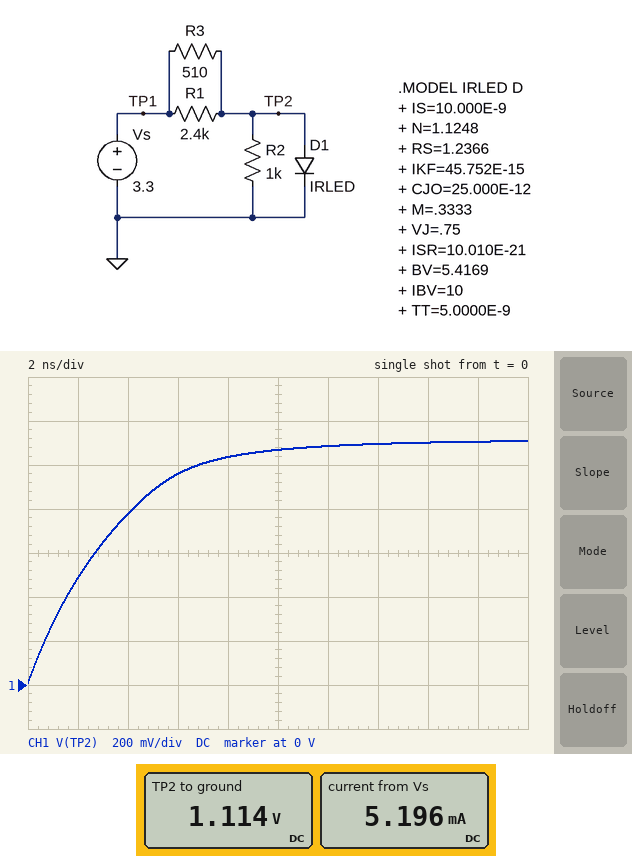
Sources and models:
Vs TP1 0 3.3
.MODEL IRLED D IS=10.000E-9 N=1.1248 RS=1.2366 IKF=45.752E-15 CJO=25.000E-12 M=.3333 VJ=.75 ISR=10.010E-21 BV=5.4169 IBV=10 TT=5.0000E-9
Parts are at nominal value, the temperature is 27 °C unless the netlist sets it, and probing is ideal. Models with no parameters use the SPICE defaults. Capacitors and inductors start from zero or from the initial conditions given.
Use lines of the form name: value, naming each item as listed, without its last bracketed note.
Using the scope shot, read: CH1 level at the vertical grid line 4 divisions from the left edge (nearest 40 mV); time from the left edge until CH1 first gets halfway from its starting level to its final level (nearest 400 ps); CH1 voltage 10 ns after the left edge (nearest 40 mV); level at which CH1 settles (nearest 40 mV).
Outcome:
CH1 level at the vertical grid line 4 divisions from the left edge: 1.04 V
time from the left edge until CH1 first gets halfway from its starting level to its final level: 2.4 ns
CH1 voltage 10 ns after the left edge: 1.08 V
level at which CH1 settles: 1.12 V
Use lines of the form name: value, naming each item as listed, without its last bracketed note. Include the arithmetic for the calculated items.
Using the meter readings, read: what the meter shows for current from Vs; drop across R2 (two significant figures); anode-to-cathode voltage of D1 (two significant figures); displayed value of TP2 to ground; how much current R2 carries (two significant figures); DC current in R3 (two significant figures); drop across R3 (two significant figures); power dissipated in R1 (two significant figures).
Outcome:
what the meter shows for current from Vs: 5.196 mA
drop across R2: 1.114 V = 1.1 V
anode-to-cathode voltage of D1: 1.114 V = 1.1 V
displayed value of TP2 to ground: 1.114 V
how much current R2 carries: (1.114 V) / 1 kΩ = 1.1 mA
DC current in R3: (3.3 V - 1.114 V) / 510 Ω = 4.3 mA
drop across R3: 3.3 V - 1.114 V = 2.2 V
power dissipated in R1: (3.3 V - 1.114 V)^2 / 2.4 kΩ = 2.0 mW
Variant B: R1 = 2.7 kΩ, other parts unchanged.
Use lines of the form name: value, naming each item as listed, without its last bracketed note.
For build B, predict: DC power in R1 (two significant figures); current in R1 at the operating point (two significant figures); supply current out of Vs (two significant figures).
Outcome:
DC power in R1: 1.8 mW
current in R1 at the operating point: 810 µA
supply current out of Vs: 5.1 mA
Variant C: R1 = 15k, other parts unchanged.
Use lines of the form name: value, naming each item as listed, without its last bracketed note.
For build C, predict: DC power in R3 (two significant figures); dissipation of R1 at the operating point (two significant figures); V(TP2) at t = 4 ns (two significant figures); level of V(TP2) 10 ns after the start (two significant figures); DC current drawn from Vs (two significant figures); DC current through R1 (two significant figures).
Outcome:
DC power in R3: 9.5 mW
dissipation of R1 at the operating point: 320 µW
V(TP2) at t = 4 ns: 700 mV
level of V(TP2) 10 ns after the start: 1.0 V
DC current drawn from Vs: 4.5 mA
DC current through R1: 150 µA
